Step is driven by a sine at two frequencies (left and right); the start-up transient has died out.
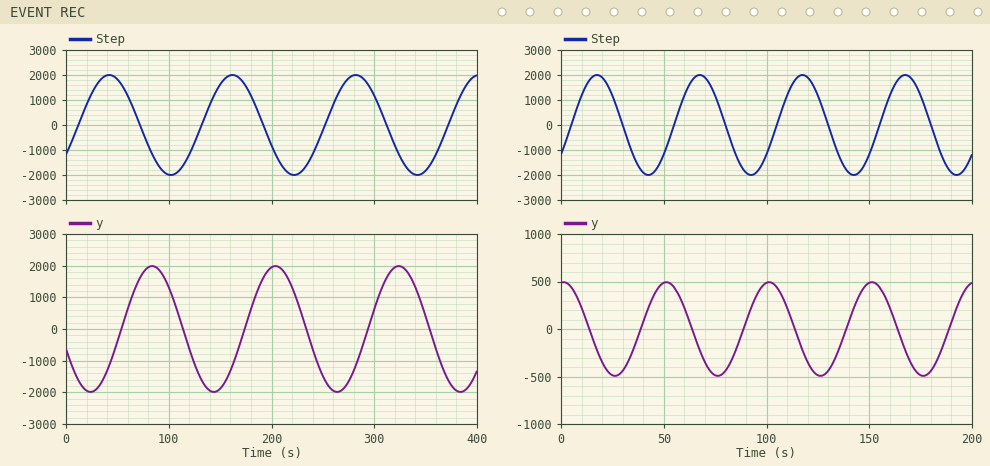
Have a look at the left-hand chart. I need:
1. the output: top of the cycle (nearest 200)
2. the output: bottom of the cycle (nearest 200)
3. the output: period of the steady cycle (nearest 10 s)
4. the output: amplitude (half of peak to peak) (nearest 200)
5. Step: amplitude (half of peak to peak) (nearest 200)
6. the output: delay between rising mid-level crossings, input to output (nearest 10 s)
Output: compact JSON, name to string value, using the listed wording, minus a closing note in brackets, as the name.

{"the output: top of the cycle": "2000", "the output: bottom of the cycle": "-2000", "the output: period of the steady cycle": "120 s", "the output: amplitude (half of peak to peak)": "2000", "Step: amplitude (half of peak to peak)": "2000", "the output: delay between rising mid-level crossings, input to output": "40 s"}
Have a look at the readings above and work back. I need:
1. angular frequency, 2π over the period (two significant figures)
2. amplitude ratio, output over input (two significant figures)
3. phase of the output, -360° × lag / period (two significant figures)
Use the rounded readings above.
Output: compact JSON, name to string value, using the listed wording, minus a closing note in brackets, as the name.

{"angular frequency, 2π over the period": "0.052 rad/s", "amplitude ratio, output over input": "1.0", "phase of the output, -360° × lag / period": "-120°"}
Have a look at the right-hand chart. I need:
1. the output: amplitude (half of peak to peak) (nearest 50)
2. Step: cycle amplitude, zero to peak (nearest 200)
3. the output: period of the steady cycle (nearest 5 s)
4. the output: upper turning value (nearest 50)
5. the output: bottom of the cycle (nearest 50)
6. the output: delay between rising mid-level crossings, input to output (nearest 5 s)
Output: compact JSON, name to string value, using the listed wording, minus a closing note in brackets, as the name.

{"the output: amplitude (half of peak to peak)": "500", "Step: cycle amplitude, zero to peak": "2000", "the output: period of the steady cycle": "50 s", "the output: upper turning value": "500", "the output: bottom of the cycle": "-500", "the output: delay between rising mid-level crossings, input to output": "35 s"}
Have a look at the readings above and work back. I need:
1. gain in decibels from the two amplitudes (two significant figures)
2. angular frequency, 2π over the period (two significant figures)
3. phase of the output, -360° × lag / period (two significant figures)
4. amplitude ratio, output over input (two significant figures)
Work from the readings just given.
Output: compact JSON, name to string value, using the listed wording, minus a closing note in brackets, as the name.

{"gain in decibels from the two amplitudes": "-12 dB", "angular frequency, 2π over the period": "0.13 rad/s", "phase of the output, -360° × lag / period": "-250°", "amplitude ratio, output over input": "0.25"}
